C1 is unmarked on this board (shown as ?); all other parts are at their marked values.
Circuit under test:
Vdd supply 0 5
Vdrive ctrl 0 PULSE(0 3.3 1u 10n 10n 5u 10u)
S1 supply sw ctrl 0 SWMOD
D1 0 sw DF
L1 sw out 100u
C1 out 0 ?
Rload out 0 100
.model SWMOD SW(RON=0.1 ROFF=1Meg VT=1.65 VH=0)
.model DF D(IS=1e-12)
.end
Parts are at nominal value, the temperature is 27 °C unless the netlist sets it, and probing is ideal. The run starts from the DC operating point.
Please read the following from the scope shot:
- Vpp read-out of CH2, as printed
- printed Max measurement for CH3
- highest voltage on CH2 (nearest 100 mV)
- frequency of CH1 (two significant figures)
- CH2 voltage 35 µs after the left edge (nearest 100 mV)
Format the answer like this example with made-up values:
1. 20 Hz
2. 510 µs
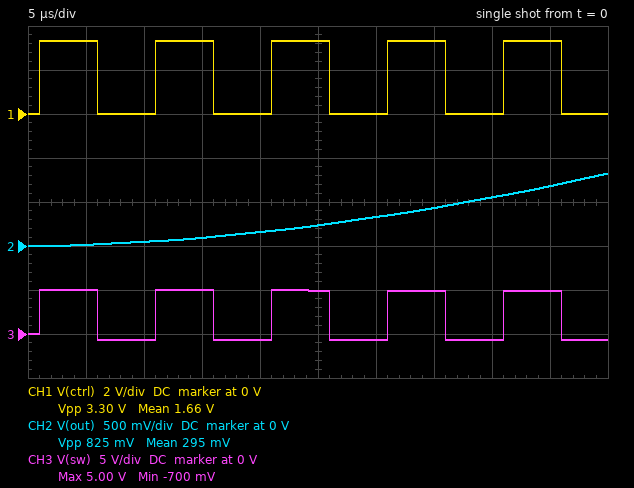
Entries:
1. 825 mV
2. 5.00 V
3. 800 mV
4. 100 kHz
5. 400 mV
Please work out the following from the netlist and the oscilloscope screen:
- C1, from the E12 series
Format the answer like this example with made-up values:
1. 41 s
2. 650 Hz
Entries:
1. 33 µF
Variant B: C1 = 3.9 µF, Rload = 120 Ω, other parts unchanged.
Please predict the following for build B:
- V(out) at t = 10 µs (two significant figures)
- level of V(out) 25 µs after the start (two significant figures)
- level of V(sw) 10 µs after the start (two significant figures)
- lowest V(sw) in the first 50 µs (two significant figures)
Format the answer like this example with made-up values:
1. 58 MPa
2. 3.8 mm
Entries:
1. 390 mV
2. 1.7 V
3. -670 mV
4. -700 mV
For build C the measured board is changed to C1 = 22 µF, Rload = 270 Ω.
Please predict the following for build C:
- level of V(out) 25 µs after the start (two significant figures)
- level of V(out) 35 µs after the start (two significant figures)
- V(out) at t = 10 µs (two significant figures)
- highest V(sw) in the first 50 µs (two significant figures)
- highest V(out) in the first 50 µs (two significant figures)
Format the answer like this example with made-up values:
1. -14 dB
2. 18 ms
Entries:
1. 350 mV
2. 640 mV
3. 72 mV
4. 5.0 V
5. 1.2 V
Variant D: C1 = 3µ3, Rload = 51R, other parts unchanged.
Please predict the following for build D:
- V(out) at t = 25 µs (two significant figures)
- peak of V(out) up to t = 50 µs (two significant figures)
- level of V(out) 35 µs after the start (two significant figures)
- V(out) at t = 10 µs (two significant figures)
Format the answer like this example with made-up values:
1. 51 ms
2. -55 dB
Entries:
1. 1.9 V
2. 3.9 V
3. 2.9 V
4. 450 mV
